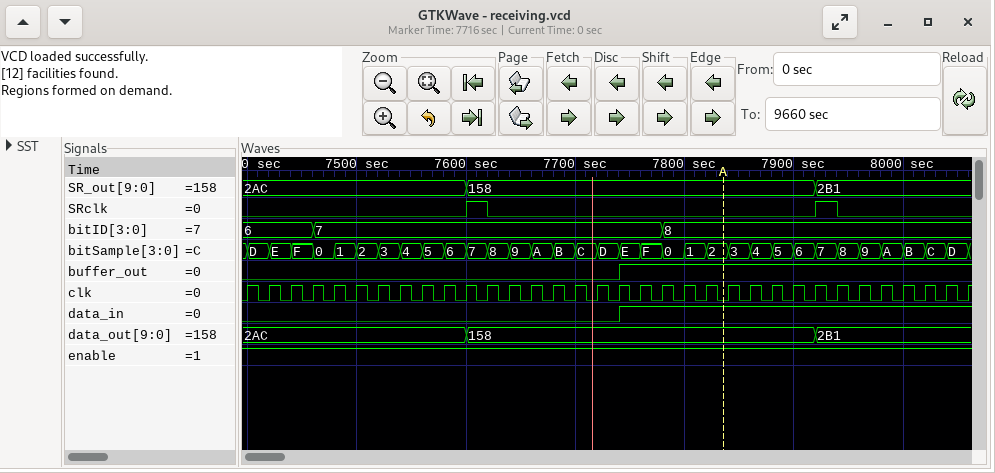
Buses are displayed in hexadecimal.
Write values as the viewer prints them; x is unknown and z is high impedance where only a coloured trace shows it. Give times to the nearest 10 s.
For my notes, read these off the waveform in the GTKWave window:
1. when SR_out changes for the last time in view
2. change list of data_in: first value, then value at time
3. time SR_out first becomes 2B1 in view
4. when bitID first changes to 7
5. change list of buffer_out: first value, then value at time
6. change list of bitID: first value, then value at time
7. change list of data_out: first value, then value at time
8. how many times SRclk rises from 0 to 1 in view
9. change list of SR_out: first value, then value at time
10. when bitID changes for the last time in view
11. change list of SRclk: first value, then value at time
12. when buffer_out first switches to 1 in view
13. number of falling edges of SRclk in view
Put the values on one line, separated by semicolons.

7920 s; 0, 1 at 7740 s; 7920 s; 7460 s; 0, 1 at 7740 s; 6, 7 at 7460 s, 8 at 7780 s; 2AC, 158 at 7600 s, 2B1 at 7920 s; 2; 2AC, 158 at 7600 s, 2B1 at 7920 s; 7780 s; 0, 1 at 7600 s, 0 at 7620 s, 1 at 7920 s, 0 at 7940 s; 7740 s; 2
